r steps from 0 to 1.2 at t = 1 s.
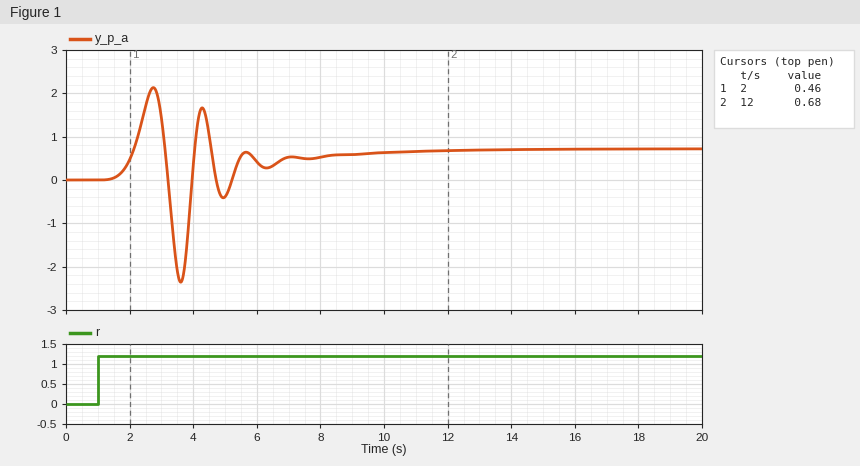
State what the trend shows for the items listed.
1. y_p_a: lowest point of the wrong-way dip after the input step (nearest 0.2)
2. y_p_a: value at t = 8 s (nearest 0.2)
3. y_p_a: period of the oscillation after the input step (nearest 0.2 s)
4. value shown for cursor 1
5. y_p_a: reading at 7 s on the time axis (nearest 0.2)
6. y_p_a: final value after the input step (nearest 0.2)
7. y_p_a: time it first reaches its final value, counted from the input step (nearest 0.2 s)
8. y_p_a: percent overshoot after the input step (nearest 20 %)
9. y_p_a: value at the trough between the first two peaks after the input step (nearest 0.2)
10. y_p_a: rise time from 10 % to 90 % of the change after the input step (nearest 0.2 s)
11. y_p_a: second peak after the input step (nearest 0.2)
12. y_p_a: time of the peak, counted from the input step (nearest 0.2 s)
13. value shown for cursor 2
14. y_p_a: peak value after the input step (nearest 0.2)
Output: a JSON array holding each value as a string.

["-2.4", "0.6", "1.6 s", "0.46", "0.6", "0.8", "1.2 s", "200 %", "-2.4", "0.6 s", "1.6", "1.8 s", "0.68", "2.2"]
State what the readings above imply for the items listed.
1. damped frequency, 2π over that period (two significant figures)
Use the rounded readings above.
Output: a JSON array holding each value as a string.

["3.9 rad/s"]
